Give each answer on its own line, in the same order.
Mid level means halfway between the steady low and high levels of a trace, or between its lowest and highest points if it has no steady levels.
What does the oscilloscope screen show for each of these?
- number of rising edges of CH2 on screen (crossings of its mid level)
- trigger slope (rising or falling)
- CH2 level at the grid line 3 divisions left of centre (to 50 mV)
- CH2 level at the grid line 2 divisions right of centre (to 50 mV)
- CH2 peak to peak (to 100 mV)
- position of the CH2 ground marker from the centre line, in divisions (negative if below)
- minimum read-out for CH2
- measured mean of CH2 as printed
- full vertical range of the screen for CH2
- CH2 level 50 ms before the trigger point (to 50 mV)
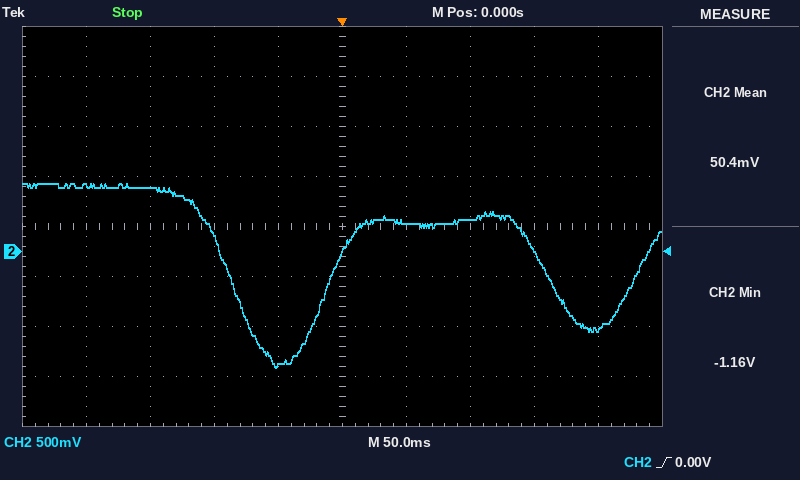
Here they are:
2
rising
650 mV
300 mV
1.80 V
-0.5 div
-1.16 V
50.4 mV
4 V
-1.15 V
